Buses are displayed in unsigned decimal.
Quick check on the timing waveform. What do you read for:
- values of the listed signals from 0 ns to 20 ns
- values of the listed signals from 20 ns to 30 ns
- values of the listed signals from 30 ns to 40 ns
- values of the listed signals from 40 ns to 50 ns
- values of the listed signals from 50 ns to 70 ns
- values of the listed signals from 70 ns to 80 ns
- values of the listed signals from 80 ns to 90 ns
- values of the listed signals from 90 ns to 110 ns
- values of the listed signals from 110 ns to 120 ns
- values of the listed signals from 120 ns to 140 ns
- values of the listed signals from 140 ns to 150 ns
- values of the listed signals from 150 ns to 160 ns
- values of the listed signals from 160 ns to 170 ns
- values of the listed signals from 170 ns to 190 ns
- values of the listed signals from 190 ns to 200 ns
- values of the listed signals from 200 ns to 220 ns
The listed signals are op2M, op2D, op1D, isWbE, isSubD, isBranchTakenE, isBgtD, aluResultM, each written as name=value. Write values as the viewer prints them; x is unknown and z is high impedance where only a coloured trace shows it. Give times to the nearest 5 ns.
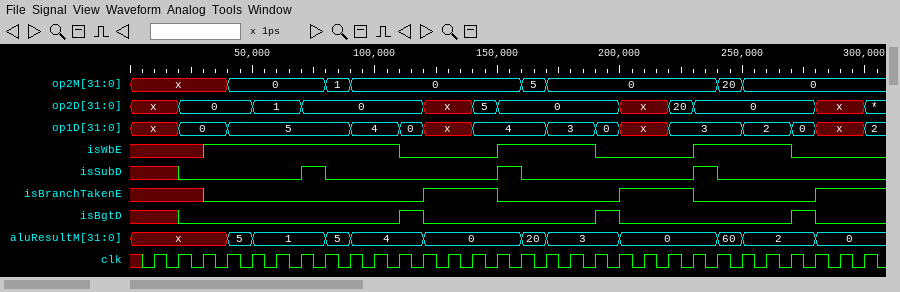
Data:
op2M=x, op2D=x, op1D=x, isWbE=x, isSubD=x, isBranchTakenE=x, isBgtD=x, aluResultM=x
op2M=x, op2D=0, op1D=0, isWbE=x, isSubD=0, isBranchTakenE=x, isBgtD=0, aluResultM=x
op2M=x, op2D=0, op1D=0, isWbE=1, isSubD=0, isBranchTakenE=0, isBgtD=0, aluResultM=x
op2M=0, op2D=0, op1D=5, isWbE=1, isSubD=0, isBranchTakenE=0, isBgtD=0, aluResultM=5
op2M=0, op2D=1, op1D=5, isWbE=1, isSubD=0, isBranchTakenE=0, isBgtD=0, aluResultM=1
op2M=0, op2D=0, op1D=5, isWbE=1, isSubD=1, isBranchTakenE=0, isBgtD=0, aluResultM=1
op2M=1, op2D=0, op1D=5, isWbE=1, isSubD=0, isBranchTakenE=0, isBgtD=0, aluResultM=5
op2M=0, op2D=0, op1D=4, isWbE=1, isSubD=0, isBranchTakenE=0, isBgtD=0, aluResultM=4
op2M=0, op2D=0, op1D=0, isWbE=0, isSubD=0, isBranchTakenE=0, isBgtD=1, aluResultM=4
op2M=0, op2D=x, op1D=x, isWbE=0, isSubD=0, isBranchTakenE=1, isBgtD=0, aluResultM=0
op2M=0, op2D=5, op1D=4, isWbE=0, isSubD=0, isBranchTakenE=1, isBgtD=0, aluResultM=0
op2M=0, op2D=0, op1D=4, isWbE=1, isSubD=1, isBranchTakenE=0, isBgtD=0, aluResultM=0
op2M=5, op2D=0, op1D=4, isWbE=1, isSubD=0, isBranchTakenE=0, isBgtD=0, aluResultM=20
op2M=0, op2D=0, op1D=3, isWbE=1, isSubD=0, isBranchTakenE=0, isBgtD=0, aluResultM=3
op2M=0, op2D=0, op1D=0, isWbE=0, isSubD=0, isBranchTakenE=0, isBgtD=1, aluResultM=3
op2M=0, op2D=x, op1D=x, isWbE=0, isSubD=0, isBranchTakenE=1, isBgtD=0, aluResultM=0
